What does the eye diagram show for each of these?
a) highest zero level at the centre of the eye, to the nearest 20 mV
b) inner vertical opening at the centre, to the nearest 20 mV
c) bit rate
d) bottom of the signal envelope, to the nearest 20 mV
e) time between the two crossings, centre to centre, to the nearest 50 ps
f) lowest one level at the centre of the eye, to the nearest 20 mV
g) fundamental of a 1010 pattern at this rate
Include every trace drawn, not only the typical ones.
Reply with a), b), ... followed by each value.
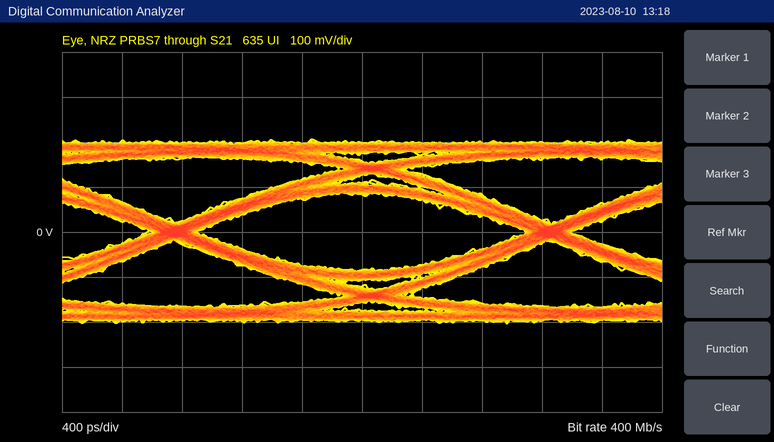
a) -80 mV
b) 160 mV
c) 400 Mb/s
d) -200 mV
e) 2.50 ns
f) 80 mV
g) 200 MHz
